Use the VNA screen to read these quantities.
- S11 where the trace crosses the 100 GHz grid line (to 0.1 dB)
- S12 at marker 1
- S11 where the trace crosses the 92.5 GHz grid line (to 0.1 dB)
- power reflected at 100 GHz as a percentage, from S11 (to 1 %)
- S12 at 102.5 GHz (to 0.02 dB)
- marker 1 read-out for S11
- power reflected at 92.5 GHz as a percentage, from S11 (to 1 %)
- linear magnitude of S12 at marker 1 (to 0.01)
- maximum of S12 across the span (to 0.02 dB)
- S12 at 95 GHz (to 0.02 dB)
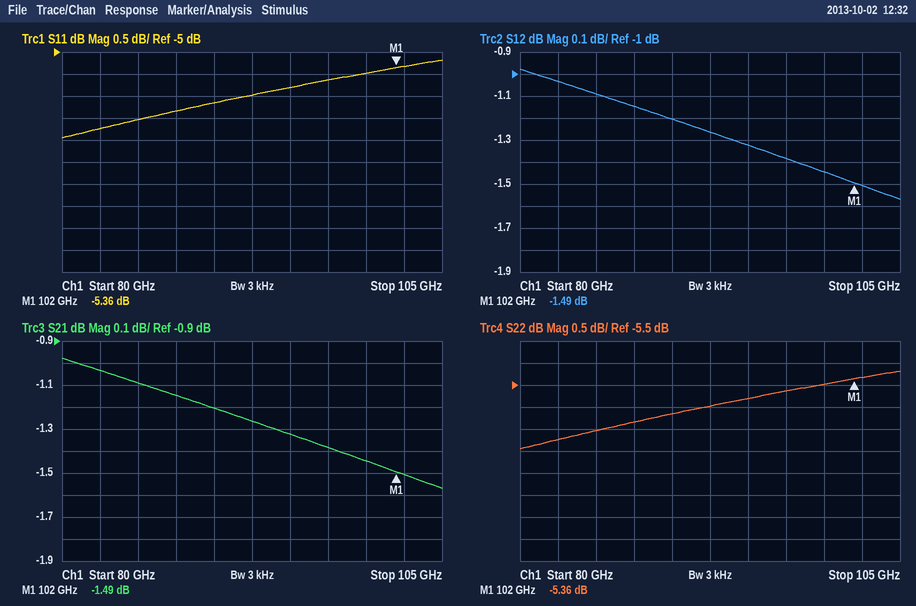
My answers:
-5.5 dB
-1.49 dB
-6.0 dB
28 %
-1.50 dB
-5.36 dB
25 %
0.84
-0.98 dB
-1.32 dB
